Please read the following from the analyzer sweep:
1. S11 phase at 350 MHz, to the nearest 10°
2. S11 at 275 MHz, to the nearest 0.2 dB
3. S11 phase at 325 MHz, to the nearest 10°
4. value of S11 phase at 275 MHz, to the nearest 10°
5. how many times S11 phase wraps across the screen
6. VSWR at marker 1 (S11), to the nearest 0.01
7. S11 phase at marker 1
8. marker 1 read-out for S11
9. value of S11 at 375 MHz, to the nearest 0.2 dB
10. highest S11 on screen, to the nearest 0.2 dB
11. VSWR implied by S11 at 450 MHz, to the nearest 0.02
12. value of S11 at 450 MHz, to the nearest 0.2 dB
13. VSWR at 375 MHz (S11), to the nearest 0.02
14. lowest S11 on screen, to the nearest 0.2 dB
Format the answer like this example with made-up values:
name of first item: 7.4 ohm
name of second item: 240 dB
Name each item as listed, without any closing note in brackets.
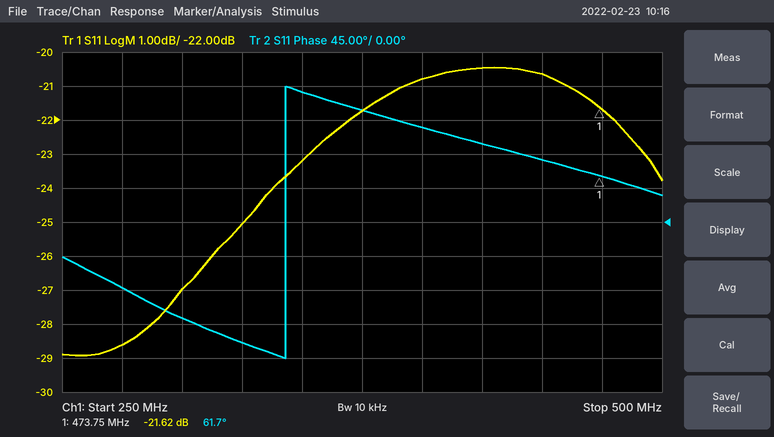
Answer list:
S11 phase at 350 MHz, to the nearest 10°: 170°
S11 at 275 MHz, to the nearest 0.2 dB: -28.6 dB
S11 phase at 325 MHz, to the nearest 10°: -160°
value of S11 phase at 275 MHz, to the nearest 10°: -90°
how many times S11 phase wraps across the screen: 1
VSWR at marker 1 (S11), to the nearest 0.01: 1.18
S11 phase at marker 1: 61.7°
marker 1 read-out for S11: -21.62 dB
value of S11 at 375 MHz, to the nearest 0.2 dB: -21.8 dB
highest S11 on screen, to the nearest 0.2 dB: -20.4 dB
VSWR implied by S11 at 450 MHz, to the nearest 0.02: 1.20
value of S11 at 450 MHz, to the nearest 0.2 dB: -20.6 dB
VSWR at 375 MHz (S11), to the nearest 0.02: 1.18
lowest S11 on screen, to the nearest 0.2 dB: -29.0 dB
